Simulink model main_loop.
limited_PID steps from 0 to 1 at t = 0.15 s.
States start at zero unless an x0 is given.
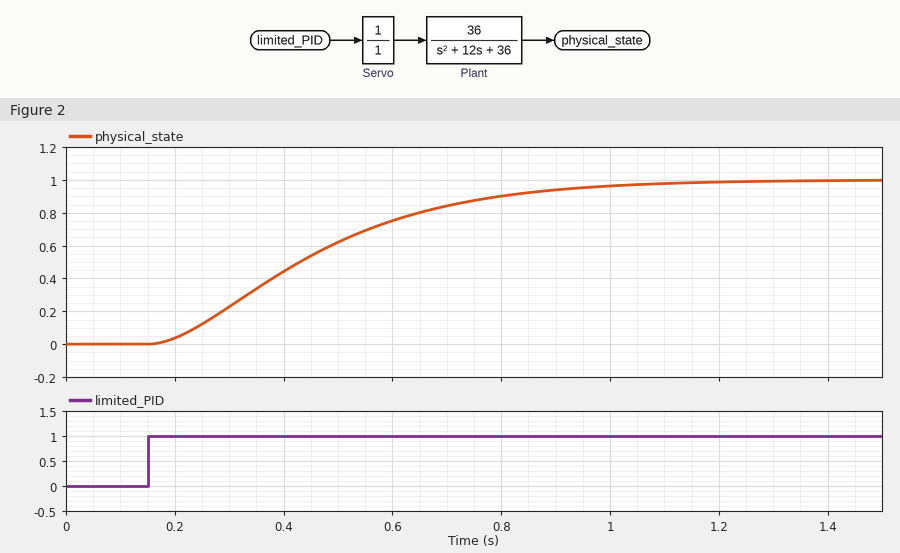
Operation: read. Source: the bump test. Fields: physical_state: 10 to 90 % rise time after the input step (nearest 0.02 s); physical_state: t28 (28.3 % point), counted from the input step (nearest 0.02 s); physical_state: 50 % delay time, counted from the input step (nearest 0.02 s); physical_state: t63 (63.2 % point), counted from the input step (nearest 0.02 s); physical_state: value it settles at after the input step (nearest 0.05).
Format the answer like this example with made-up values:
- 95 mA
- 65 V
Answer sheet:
- 0.56 s
- 0.18 s
- 0.28 s
- 0.36 s
- 1.00
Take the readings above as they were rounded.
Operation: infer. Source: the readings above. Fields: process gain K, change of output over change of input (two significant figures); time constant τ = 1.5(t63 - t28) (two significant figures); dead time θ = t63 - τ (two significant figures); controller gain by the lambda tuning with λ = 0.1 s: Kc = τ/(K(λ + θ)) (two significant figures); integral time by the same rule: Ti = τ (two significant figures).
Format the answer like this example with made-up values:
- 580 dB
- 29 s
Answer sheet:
- 1.0
- 0.27 s
- 0.090 s
- 1.4
- 0.27 s
